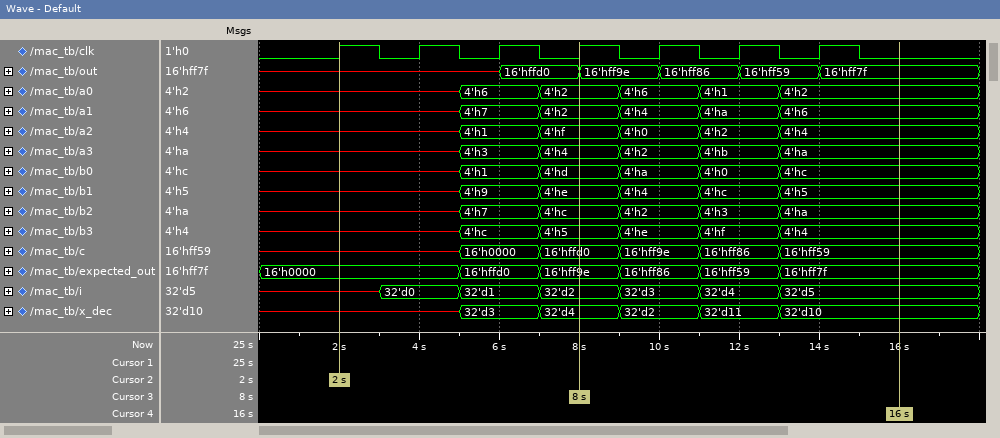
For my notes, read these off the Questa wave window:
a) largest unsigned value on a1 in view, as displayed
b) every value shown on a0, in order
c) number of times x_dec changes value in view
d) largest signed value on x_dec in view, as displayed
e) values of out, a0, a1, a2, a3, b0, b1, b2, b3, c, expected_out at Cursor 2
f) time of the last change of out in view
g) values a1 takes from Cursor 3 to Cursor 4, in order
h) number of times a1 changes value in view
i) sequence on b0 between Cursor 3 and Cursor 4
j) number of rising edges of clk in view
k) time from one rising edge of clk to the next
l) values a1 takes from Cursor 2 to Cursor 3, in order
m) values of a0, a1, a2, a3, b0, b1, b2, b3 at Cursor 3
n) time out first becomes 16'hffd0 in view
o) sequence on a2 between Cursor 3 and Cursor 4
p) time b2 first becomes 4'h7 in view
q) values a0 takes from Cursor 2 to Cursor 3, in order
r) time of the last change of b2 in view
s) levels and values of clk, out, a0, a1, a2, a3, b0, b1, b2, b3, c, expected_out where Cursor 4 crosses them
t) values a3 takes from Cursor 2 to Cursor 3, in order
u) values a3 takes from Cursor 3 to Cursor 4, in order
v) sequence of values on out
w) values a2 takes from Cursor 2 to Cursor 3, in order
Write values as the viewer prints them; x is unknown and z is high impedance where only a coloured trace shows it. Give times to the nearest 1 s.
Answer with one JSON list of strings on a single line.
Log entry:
["4'ha", "x, 4'h6, 4'h2, 4'h6, 4'h1, 4'h2", "5", "32'd11", "out=x, a0=x, a1=x, a2=x, a3=x, b0=x, b1=x, b2=x, b3=x, c=x, expected_out=16'h0000", "14 s", "4'h2, 4'h4, 4'ha, 4'h6", "5", "4'hd, 4'ha, 4'h0, 4'hc", "7", "2 s", "x, 4'h7, 4'h2", "a0=4'h2, a1=4'h2, a2=4'hf, a3=4'h4, b0=4'hd, b1=4'he, b2=4'hc, b3=4'h5", "6 s", "4'hf, 4'h0, 4'h2, 4'h4", "5 s", "x, 4'h6, 4'h2", "13 s", "clk=0, out=16'hff7f, a0=4'h2, a1=4'h6, a2=4'h4, a3=4'ha, b0=4'hc, b1=4'h5, b2=4'ha, b3=4'h4, c=16'hff59, expected_out=16'hff7f", "x, 4'h3, 4'h4", "4'h4, 4'h2, 4'hb, 4'ha", "x, 16'hffd0, 16'hff9e, 16'hff86, 16'hff59, 16'hff7f", "x, 4'h1, 4'hf"]
